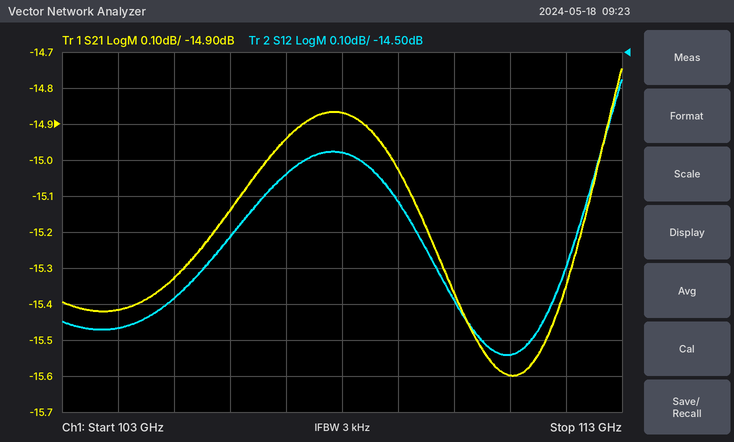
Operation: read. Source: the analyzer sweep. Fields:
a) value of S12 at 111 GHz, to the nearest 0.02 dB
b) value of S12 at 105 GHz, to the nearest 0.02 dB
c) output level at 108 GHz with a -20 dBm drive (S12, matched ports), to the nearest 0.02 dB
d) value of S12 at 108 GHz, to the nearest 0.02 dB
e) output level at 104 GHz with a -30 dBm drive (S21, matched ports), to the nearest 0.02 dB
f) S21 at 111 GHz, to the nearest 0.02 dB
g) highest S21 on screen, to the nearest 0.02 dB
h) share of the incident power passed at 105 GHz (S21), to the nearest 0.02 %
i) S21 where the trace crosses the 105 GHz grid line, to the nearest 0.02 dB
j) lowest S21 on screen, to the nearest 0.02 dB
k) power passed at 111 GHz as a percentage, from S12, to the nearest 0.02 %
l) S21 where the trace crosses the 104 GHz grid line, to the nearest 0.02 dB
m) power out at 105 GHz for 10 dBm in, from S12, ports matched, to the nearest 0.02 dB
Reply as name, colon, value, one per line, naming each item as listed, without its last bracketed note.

value of S12 at 111 GHz, to the nearest 0.02 dB: -15.34 dB
value of S12 at 105 GHz, to the nearest 0.02 dB: -15.18 dB
output level at 108 GHz with a -20 dBm drive (S12, matched ports), to the nearest 0.02 dB: -34.78 dBm
value of S12 at 108 GHz, to the nearest 0.02 dB: -14.78 dB
output level at 104 GHz with a -30 dBm drive (S21, matched ports), to the nearest 0.02 dB: -45.42 dBm
S21 at 111 GHz, to the nearest 0.02 dB: -15.60 dB
highest S21 on screen, to the nearest 0.02 dB: -14.74 dB
share of the incident power passed at 105 GHz (S21), to the nearest 0.02 %: 2.94 %
S21 where the trace crosses the 105 GHz grid line, to the nearest 0.02 dB: -15.32 dB
lowest S21 on screen, to the nearest 0.02 dB: -15.60 dB
power passed at 111 GHz as a percentage, from S12, to the nearest 0.02 %: 2.92 %
S21 where the trace crosses the 104 GHz grid line, to the nearest 0.02 dB: -15.42 dB
power out at 105 GHz for 10 dBm in, from S12, ports matched, to the nearest 0.02 dB: -5.18 dBm
